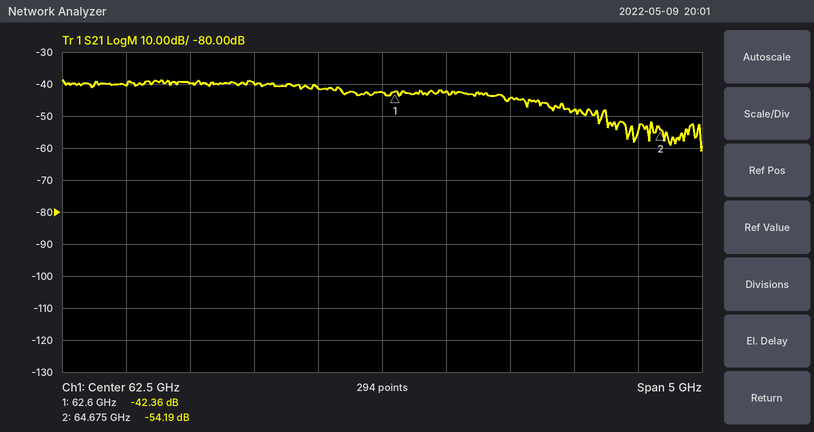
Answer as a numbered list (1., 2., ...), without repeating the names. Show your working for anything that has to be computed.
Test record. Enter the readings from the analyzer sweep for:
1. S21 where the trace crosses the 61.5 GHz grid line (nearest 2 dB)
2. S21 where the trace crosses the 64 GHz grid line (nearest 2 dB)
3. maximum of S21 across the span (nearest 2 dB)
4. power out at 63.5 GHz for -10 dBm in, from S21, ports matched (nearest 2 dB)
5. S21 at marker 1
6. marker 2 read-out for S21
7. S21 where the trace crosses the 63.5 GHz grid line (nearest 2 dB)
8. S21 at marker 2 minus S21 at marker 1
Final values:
1. -40 dB
2. -48 dB
3. -38 dB
4. -10 dBm + (-44 dB) = -54 dBm
5. -42.36 dB
6. -54.19 dB
7. -44 dB
8. -54.19 − (-42.36) = -11.83 dB
